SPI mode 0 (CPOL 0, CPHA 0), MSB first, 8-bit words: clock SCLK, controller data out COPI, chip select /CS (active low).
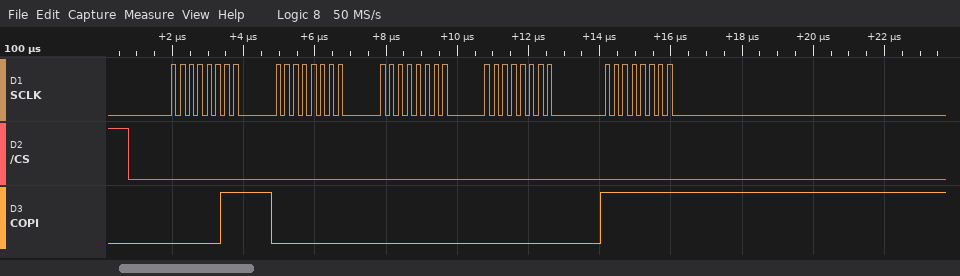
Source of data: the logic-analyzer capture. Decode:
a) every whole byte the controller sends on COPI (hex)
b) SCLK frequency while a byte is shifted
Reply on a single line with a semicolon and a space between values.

0x03 0x00 0x00 0x00 0xFF; 4 MHz
